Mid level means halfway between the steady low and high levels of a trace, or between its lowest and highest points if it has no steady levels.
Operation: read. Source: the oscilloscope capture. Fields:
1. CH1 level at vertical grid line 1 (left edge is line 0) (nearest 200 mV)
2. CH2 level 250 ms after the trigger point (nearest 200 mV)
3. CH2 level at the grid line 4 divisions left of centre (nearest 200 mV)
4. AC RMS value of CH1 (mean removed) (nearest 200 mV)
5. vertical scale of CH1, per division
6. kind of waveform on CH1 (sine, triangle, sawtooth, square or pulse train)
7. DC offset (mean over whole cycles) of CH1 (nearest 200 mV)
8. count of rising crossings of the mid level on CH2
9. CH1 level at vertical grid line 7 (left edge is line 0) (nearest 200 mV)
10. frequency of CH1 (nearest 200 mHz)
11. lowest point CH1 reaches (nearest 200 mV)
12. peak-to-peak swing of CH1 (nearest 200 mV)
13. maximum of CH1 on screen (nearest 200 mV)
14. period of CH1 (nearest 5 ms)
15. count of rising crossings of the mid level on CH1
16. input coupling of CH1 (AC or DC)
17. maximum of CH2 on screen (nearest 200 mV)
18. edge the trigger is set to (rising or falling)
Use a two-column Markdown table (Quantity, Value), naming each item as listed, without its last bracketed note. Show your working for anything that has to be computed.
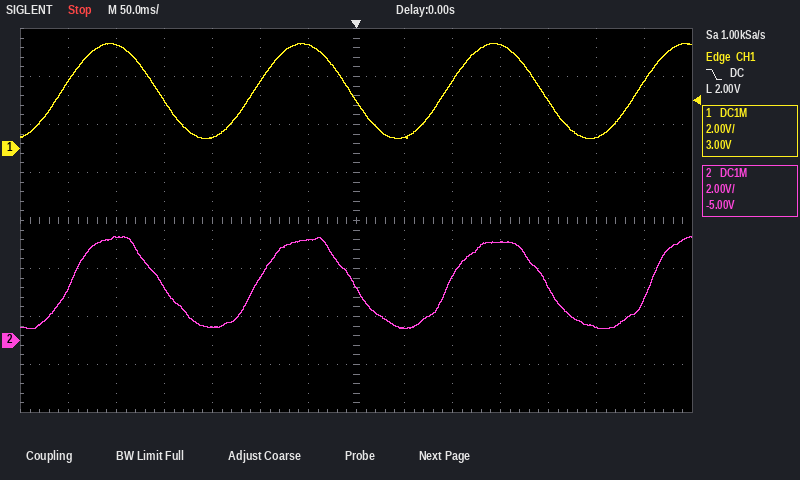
| Quantity | Value |
|---|---|
| CH1 level at vertical grid line 1 (left edge is line 0) | 2.8 V |
| CH2 level 250 ms after the trigger point | 600 mV |
| CH2 level at the grid line 4 divisions left of centre | 2.2 V |
| AC RMS value of CH1 (mean removed) | 4.0 V / (2√2) ≈ 1.4 V |
| vertical scale of CH1, per division | 2 V |
| kind of waveform on CH1 | sine |
| DC offset (mean over whole cycles) of CH1 | (4.4 V + (400 mV)) / 2 ≈ 2.4 V |
| count of rising crossings of the mid level on CH2 | 4 |
| CH1 level at vertical grid line 7 (left edge is line 0) | 2.0 V |
| frequency of CH1 | 1 / 200 ms ≈ 5.0 Hz |
| lowest point CH1 reaches | 400 mV |
| peak-to-peak swing of CH1 | 4.4 V − (400 mV) = 4.0 V |
| maximum of CH1 on screen | 4.4 V |
| period of CH1 | 200 ms |
| count of rising crossings of the mid level on CH1 | 4 |
| input coupling of CH1 | DC |
| maximum of CH2 on screen | 4.4 V |
| edge the trigger is set to | falling |
